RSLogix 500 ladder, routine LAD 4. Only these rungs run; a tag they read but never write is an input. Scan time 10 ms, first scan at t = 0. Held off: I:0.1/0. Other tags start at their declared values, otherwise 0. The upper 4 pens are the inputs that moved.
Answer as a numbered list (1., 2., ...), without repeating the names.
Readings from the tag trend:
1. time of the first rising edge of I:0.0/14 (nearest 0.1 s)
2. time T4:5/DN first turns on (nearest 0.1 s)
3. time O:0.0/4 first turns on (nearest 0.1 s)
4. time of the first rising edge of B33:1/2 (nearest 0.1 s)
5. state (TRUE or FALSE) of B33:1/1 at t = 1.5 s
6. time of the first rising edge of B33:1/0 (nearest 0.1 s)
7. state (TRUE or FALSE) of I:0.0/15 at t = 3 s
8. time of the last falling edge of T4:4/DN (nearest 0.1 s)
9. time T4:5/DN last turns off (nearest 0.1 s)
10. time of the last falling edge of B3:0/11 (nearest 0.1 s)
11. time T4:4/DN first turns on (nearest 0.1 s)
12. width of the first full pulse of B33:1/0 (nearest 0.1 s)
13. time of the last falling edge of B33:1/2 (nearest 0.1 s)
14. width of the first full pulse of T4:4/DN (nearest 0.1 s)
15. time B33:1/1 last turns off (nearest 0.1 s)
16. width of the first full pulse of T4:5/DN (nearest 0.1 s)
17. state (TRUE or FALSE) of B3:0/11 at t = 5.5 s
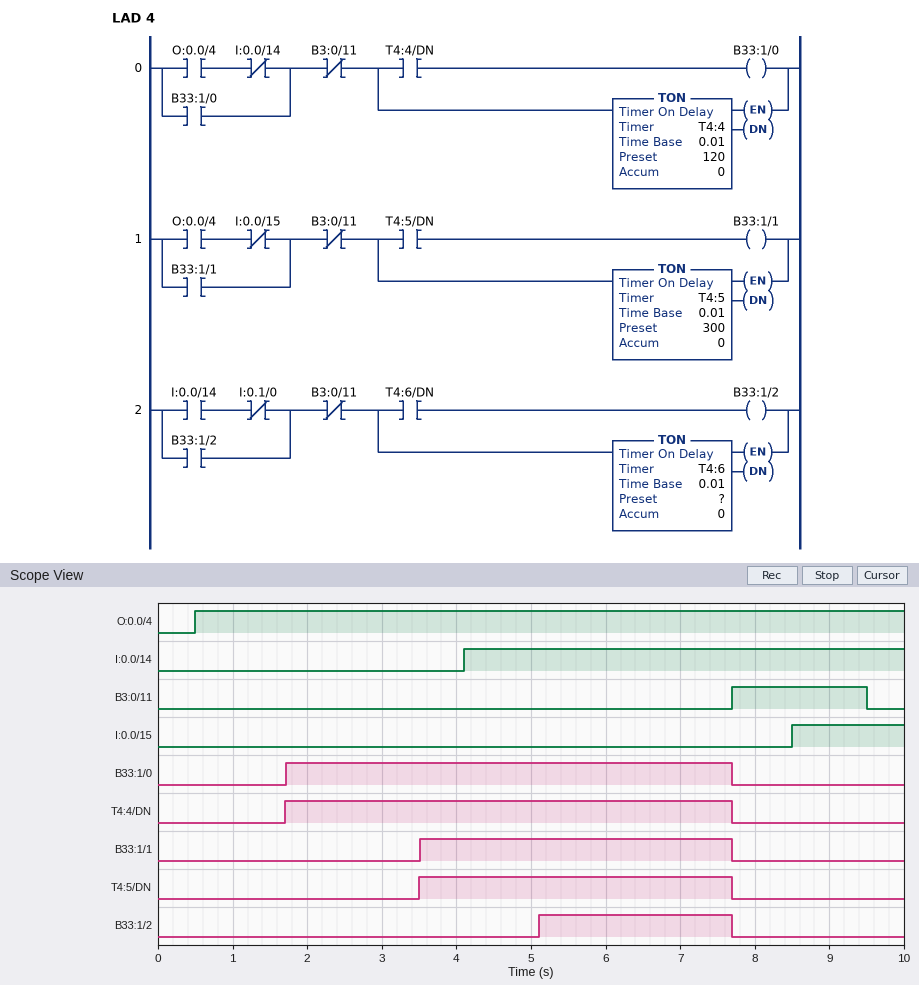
1. 4.1 s
2. 3.5 s
3. 0.5 s
4. 5.1 s
5. FALSE
6. 1.7 s
7. FALSE
8. 7.7 s
9. 7.7 s
10. 9.5 s
11. 1.7 s
12. 6.0 s
13. 7.7 s
14. 6.0 s
15. 7.7 s
16. 4.2 s
17. FALSE
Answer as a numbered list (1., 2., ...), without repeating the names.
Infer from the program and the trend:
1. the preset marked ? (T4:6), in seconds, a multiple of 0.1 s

1. 1.0 s
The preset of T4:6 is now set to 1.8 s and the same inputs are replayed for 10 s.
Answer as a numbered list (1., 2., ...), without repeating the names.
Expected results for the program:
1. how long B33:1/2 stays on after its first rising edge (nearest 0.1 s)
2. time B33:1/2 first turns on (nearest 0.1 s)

1. 1.8 s
2. 5.9 s
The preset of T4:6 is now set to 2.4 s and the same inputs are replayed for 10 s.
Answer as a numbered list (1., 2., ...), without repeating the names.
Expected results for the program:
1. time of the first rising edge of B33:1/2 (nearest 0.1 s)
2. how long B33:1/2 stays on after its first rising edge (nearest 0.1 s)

1. 6.5 s
2. 1.2 s
